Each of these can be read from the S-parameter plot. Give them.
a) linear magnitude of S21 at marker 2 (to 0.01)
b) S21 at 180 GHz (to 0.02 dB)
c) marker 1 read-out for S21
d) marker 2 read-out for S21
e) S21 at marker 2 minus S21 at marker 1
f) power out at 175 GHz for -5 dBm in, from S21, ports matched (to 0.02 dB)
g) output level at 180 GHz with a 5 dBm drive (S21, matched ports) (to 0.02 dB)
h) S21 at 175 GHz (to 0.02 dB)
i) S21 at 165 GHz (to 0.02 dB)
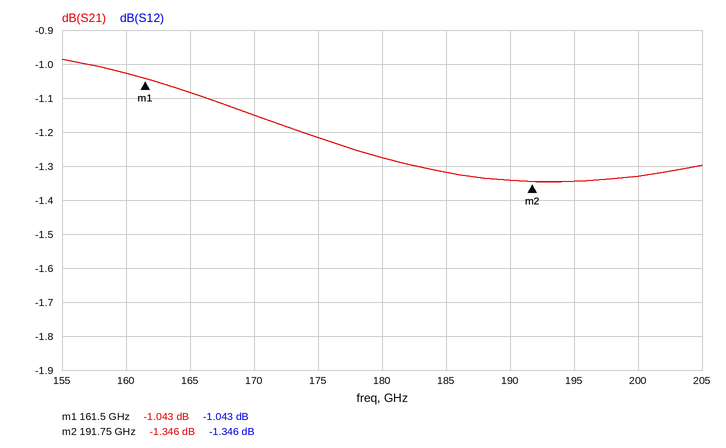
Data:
0.86
-1.28 dB
-1.043 dB
-1.346 dB
-0.303 dB
-6.22 dBm
3.72 dBm
-1.22 dB
-1.08 dB
